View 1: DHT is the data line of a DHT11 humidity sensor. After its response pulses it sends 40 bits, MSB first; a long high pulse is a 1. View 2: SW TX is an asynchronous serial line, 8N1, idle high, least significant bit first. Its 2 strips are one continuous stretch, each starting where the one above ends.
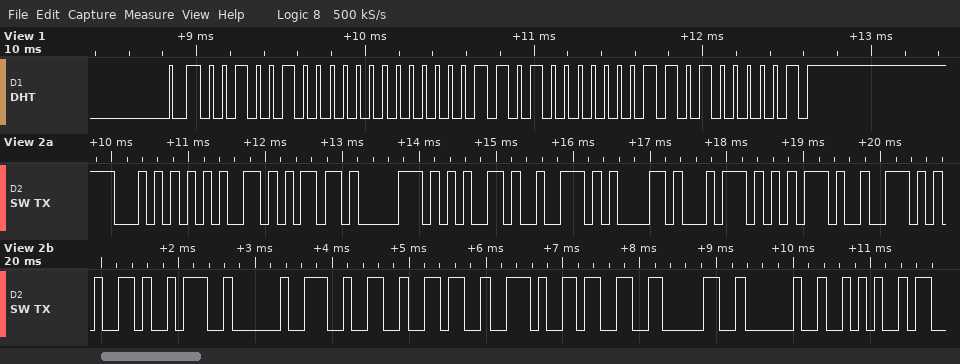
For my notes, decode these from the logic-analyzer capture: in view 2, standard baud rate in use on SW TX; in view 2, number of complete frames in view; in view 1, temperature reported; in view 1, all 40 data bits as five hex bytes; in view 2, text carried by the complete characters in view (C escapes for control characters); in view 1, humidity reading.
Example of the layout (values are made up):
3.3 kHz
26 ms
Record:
9600 baud
20
26.3 °C
24 00 1A 03 41
"Temperature: 26.30 *"
36 %
